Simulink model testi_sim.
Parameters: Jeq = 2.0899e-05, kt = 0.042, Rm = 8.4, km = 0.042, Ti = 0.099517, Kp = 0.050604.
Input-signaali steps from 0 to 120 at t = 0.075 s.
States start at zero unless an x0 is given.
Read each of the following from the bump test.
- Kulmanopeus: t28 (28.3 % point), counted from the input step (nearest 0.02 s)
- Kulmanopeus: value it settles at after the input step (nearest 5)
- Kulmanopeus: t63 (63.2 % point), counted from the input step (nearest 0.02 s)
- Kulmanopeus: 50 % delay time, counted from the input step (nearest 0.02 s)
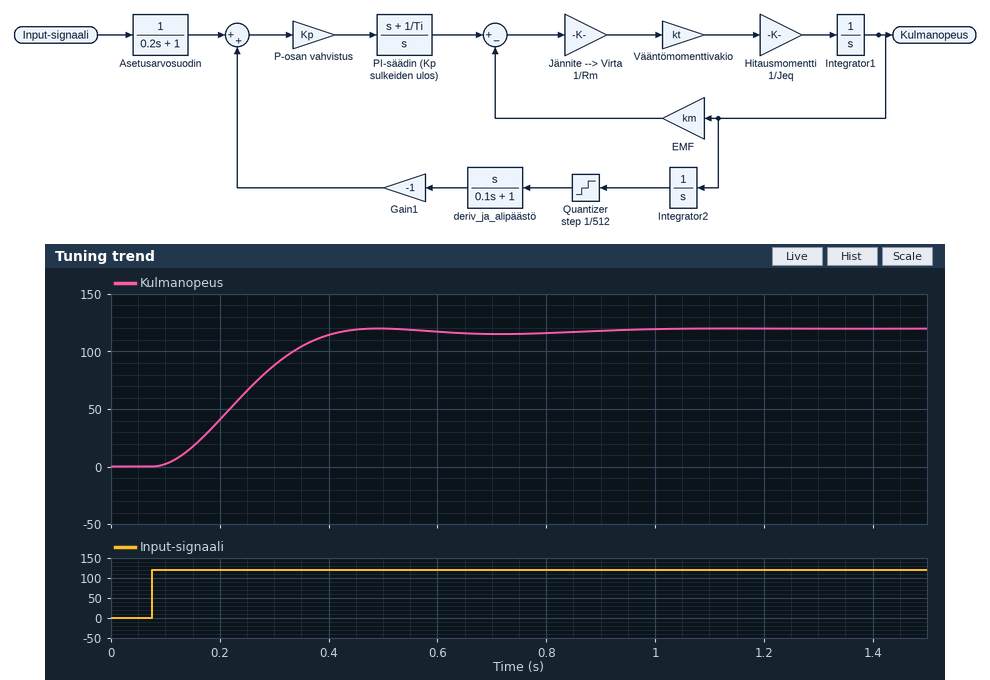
0.12 s
120
0.20 s
0.16 s
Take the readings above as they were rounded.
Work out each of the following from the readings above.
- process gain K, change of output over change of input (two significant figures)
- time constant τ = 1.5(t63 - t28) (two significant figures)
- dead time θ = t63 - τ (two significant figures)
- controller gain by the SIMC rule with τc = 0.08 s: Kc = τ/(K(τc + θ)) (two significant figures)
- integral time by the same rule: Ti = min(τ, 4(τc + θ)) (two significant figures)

1.0
0.12 s
0.080 s
0.75
0.12 s
